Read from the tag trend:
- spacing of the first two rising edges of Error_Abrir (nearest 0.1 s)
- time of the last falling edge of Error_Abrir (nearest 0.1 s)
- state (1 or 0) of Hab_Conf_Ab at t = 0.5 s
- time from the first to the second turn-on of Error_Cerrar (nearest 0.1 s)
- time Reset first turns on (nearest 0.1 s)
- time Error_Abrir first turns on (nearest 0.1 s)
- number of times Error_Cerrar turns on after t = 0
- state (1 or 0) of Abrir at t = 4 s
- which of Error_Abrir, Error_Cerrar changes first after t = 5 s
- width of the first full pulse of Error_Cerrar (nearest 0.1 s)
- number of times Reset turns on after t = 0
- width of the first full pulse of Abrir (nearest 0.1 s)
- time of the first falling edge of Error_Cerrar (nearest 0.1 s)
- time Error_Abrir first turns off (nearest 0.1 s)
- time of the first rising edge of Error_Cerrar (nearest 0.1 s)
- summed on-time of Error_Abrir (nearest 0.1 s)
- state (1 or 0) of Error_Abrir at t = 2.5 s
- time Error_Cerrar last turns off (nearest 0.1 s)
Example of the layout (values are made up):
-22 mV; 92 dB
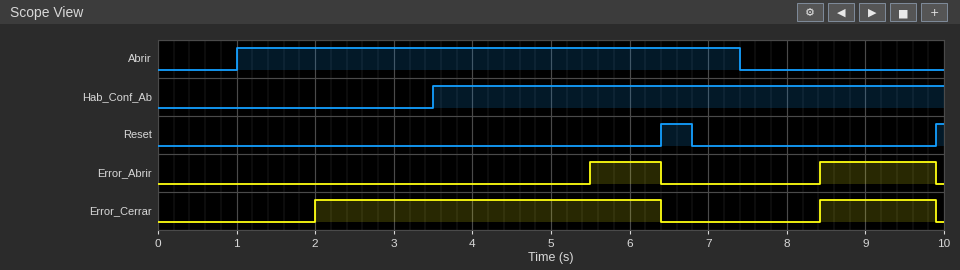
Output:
2.9 s; 9.9 s; 0; 6.4 s; 6.4 s; 5.5 s; 2; 1; Error_Abrir; 4.4 s; 2; 6.4 s; 6.4 s; 6.4 s; 2.0 s; 2.4 s; 0; 9.9 s
